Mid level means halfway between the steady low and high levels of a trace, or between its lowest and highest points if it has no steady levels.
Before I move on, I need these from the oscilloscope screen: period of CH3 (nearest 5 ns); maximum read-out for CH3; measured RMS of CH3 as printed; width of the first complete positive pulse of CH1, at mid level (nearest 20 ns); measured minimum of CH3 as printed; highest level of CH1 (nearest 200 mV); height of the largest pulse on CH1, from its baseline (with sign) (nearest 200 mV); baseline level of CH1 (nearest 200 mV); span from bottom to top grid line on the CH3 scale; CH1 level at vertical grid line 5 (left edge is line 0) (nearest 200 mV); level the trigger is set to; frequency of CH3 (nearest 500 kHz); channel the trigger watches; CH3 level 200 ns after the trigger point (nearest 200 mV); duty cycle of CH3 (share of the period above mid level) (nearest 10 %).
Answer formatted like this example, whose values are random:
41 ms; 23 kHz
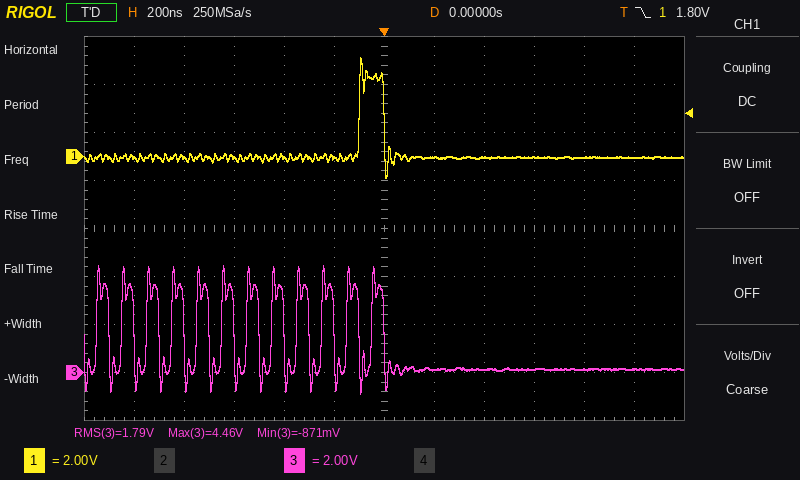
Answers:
100 ns; 4.46 V; 1.79 V; 100 ns; -871 mV; 4.2 V; +4.2 V; 0.0 V; 16 V; 0.0 V; 1.80 V; 10.0 MHz; CH1; 200 mV; 50 %
